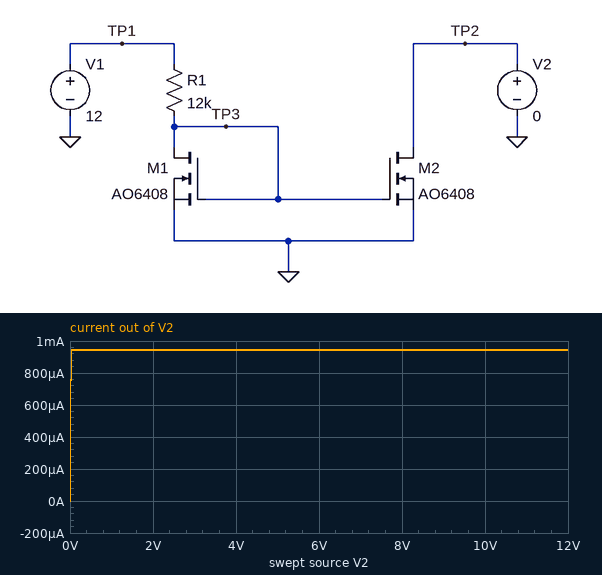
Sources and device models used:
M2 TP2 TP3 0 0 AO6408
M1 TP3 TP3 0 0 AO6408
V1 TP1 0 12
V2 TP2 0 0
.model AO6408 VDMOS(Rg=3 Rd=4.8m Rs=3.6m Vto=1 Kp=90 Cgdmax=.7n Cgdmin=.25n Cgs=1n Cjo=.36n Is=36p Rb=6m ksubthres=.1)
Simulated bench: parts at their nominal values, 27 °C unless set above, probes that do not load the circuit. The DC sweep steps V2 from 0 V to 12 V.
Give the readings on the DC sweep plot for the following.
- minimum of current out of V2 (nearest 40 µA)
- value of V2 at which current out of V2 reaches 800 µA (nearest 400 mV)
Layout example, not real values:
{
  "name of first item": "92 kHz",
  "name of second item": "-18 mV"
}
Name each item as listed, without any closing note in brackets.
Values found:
{
  "minimum of current out of V2": "0 A",
  "value of V2 at which current out of V2 reaches 800 µA": "0 V"
}
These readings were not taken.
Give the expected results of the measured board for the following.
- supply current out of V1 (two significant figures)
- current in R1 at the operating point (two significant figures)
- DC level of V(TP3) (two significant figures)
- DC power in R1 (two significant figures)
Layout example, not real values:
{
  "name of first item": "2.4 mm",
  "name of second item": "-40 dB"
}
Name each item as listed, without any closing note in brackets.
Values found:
{
  "supply current out of V1": "940 µA",
  "current in R1 at the operating point": "940 µA",
  "DC level of V(TP3)": "690 mV",
  "DC power in R1": "11 mW"
}
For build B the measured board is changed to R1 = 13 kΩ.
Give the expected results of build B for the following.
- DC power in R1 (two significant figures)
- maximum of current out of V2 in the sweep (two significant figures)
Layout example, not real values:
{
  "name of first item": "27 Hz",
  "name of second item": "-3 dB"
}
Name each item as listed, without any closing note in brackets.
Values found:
{
  "DC power in R1": "9.8 mW",
  "maximum of current out of V2 in the sweep": "870 µA"
}
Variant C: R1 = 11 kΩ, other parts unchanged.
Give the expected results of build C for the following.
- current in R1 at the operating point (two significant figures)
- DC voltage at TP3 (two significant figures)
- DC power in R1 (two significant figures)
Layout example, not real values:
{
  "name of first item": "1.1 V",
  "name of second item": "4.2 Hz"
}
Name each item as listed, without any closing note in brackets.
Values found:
{
  "current in R1 at the operating point": "1.0 mA",
  "DC voltage at TP3": "700 mV",
  "DC power in R1": "12 mW"
}
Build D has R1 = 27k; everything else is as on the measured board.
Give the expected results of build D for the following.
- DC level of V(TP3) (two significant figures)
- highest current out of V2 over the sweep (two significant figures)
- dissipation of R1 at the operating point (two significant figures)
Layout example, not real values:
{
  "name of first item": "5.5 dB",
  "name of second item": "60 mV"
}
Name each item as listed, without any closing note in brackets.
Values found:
{
  "DC level of V(TP3)": "650 mV",
  "highest current out of V2 over the sweep": "420 µA",
  "dissipation of R1 at the operating point": "4.8 mW"
}
